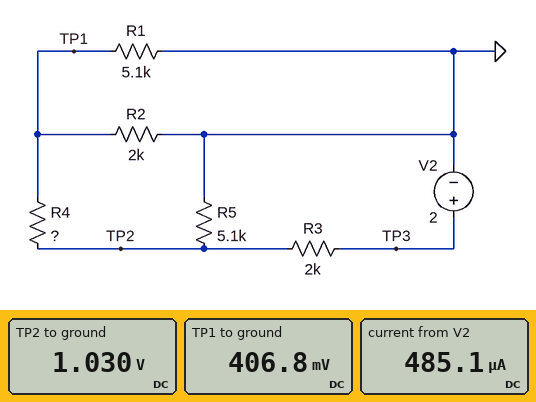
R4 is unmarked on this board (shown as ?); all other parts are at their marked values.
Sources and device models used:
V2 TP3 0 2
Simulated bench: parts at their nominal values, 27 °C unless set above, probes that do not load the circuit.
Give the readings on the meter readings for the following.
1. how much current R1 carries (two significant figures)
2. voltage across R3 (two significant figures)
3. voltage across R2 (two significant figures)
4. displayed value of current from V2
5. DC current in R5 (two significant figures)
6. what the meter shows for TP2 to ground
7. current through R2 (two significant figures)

80 µA
970 mV
410 mV
485.1 µA
200 µA
1.030 V
200 µA
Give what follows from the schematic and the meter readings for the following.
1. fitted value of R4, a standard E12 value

2.2 kΩ
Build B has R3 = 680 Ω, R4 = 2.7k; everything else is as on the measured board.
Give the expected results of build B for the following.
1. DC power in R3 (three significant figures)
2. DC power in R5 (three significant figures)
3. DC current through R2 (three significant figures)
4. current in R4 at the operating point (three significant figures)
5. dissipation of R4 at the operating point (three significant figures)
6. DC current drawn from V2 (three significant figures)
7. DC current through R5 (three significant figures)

310 µW
466 µW
268 µA
373 µA
375 µW
675 µA
302 µA
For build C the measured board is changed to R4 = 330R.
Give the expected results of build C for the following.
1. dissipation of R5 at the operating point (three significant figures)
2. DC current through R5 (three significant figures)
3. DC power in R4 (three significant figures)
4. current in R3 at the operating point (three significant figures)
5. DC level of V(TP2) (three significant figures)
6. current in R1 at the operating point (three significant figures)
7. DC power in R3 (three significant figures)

123 µW
155 µA
66.4 µW
604 µA
792 mV
126 µA
729 µW
